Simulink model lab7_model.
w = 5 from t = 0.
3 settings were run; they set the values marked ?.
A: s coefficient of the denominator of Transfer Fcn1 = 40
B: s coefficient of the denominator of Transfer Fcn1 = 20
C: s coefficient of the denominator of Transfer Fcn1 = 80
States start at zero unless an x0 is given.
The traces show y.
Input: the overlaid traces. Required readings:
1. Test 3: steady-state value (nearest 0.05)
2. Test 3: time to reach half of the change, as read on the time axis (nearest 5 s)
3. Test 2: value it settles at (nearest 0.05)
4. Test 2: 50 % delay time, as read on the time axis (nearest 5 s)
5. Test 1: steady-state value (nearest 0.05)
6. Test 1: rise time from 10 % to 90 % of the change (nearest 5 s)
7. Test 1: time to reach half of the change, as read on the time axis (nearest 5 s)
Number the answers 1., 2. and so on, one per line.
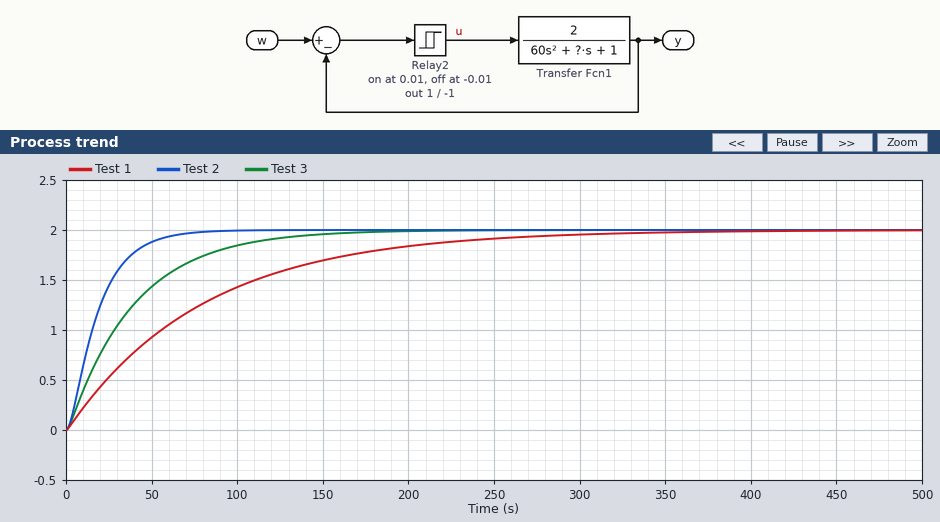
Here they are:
1. 2.00
2. 30 s
3. 2.00
4. 15 s
5. 2.00
6. 175 s
7. 55 s
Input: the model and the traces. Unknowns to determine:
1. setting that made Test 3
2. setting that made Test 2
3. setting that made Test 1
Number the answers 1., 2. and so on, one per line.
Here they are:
1. A
2. B
3. C
